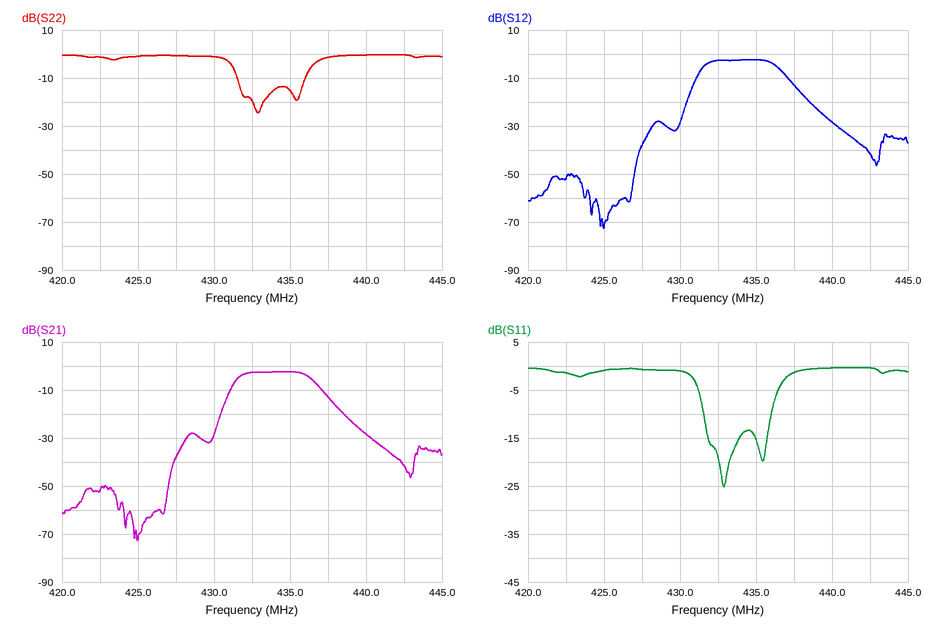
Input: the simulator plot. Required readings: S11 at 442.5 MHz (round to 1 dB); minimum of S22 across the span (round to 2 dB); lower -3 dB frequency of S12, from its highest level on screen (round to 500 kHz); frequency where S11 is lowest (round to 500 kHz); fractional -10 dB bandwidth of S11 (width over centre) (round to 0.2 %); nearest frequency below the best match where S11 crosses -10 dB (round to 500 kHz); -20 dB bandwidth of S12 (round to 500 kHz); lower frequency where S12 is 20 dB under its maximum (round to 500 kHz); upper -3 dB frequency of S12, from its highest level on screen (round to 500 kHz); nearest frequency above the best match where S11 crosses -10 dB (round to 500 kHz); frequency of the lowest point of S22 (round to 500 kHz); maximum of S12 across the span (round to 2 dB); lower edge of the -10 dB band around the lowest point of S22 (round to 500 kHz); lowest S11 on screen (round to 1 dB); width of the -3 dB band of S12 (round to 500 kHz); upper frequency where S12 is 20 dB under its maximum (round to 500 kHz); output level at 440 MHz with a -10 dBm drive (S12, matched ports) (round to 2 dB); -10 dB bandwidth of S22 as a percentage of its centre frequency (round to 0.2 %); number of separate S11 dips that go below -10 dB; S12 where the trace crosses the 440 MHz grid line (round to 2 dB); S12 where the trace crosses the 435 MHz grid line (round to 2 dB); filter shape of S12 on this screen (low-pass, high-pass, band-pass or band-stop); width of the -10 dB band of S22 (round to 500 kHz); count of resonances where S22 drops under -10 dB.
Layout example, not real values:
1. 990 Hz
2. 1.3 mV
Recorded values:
1. 0 dB
2. -24 dB
3. 431.5 MHz
4. 433.0 MHz
5. 1.0 %
6. 431.5 MHz
7. 8.5 MHz
8. 430.5 MHz
9. 436.5 MHz
10. 436.0 MHz
11. 433.0 MHz
12. -2 dB
13. 431.5 MHz
14. -25 dB
15. 5.0 MHz
16. 439.0 MHz
17. -38 dBm
18. 1.0 %
19. 2
20. -28 dB
21. -2 dB
22. band-pass
23. 4.5 MHz
24. 2
